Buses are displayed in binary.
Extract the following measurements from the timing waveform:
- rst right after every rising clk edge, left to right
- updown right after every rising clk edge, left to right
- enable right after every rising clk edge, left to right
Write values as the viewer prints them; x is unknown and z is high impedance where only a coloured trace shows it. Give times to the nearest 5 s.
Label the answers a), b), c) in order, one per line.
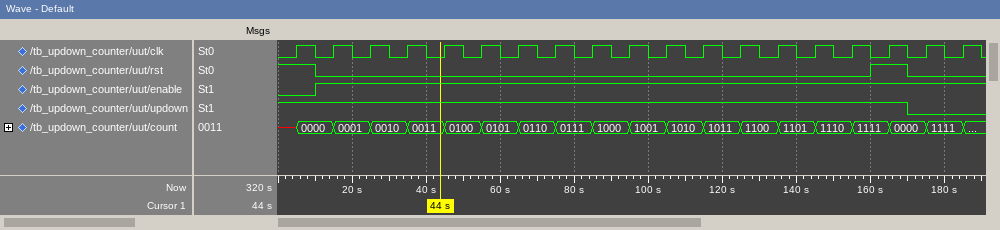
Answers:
a) 1 0 0 0 0 0 0 0 0 0 0 0 0 0 0 0 1 0 0
b) 1 1 1 1 1 1 1 1 1 1 1 1 1 1 1 1 1 0 0
c) 0 1 1 1 1 1 1 1 1 1 1 1 1 1 1 1 1 1 1
